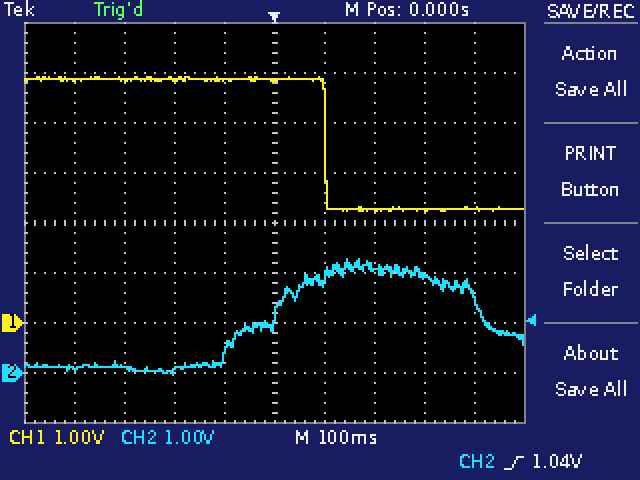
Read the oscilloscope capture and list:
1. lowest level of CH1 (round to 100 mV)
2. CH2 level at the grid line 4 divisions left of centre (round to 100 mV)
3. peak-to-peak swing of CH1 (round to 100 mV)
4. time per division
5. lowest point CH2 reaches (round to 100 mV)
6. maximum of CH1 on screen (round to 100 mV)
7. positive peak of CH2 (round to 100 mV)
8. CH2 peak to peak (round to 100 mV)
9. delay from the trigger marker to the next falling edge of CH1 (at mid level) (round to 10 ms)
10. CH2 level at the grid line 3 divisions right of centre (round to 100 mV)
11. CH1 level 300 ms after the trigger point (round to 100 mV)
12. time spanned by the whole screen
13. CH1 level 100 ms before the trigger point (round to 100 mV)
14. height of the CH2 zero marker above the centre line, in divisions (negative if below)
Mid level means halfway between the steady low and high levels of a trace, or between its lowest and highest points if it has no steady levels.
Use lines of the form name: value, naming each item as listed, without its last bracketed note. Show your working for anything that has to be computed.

lowest level of CH1: 2.2 V
CH2 level at the grid line 4 divisions left of centre: 100 mV
peak-to-peak swing of CH1: 4.9 V − (2.2 V) = 2.7 V
time per division: 100 ms
lowest point CH2 reaches: 0.0 V
maximum of CH1 on screen: 4.9 V
positive peak of CH2: 2.3 V
CH2 peak to peak: 2.3 V − (0.0 V) = 2.3 V
delay from the trigger marker to the next falling edge of CH1 (at mid level): 100 ms
CH2 level at the grid line 3 divisions right of centre: 1.9 V
CH1 level 300 ms after the trigger point: 2.3 V
time spanned by the whole screen: 1 s
CH1 level 100 ms before the trigger point: 4.9 V
height of the CH2 zero marker above the centre line, in divisions: -3.0 div
